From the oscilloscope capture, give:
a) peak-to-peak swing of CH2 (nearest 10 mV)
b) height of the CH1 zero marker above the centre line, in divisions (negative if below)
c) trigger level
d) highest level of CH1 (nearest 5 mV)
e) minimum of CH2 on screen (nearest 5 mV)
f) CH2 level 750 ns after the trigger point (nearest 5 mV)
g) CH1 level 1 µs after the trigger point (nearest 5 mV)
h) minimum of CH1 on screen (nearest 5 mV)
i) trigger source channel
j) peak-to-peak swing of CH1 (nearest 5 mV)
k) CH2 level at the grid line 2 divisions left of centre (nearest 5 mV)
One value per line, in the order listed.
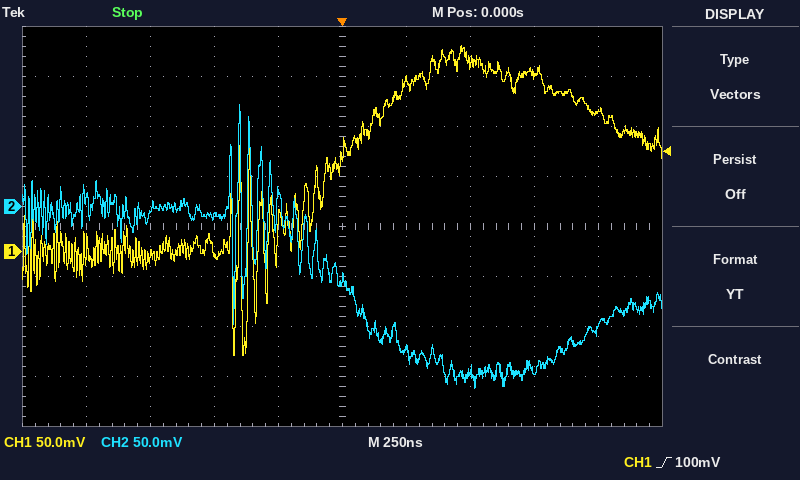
280 mV
-0.5 div
100 mV
205 mV
-180 mV
-165 mV
140 mV
-105 mV
CH1
310 mV
-10 mV
